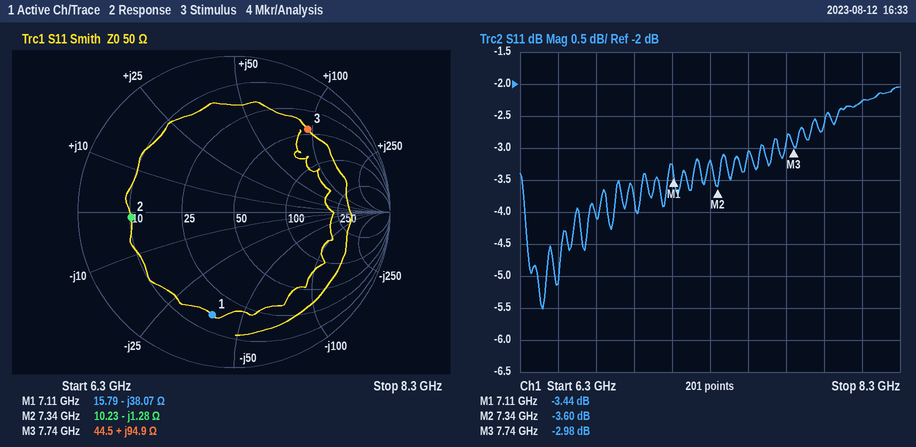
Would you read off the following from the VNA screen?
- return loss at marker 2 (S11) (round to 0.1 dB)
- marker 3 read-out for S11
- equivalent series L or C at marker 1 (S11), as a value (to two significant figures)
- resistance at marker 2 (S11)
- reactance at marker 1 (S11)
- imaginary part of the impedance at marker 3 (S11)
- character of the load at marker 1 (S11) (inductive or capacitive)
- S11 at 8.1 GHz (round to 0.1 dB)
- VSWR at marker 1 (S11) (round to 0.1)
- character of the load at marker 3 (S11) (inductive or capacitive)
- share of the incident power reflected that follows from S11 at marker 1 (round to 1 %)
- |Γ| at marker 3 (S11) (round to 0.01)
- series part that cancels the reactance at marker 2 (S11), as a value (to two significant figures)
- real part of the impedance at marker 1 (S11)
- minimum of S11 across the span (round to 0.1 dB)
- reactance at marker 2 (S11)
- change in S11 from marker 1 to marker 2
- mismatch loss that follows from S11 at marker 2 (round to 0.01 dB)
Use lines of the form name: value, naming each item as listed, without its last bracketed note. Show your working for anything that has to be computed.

return loss at marker 2 (S11): 3.6 dB
marker 3 read-out for S11: -2.98 dB
equivalent series L or C at marker 1 (S11), as a value: C = 1/(2π × 7.11 GHz × 38.07 Ω) ≈ 588 fF, so 590 fF to two significant figures
resistance at marker 2: 10.23 Ω
reactance at marker 1: -38.07 Ω
imaginary part of the impedance at marker 3: +94.9 Ω
character of the load at marker 1 (S11): capacitive
S11 at 8.1 GHz: -2.3 dB
VSWR at marker 1 (S11): 5.1
character of the load at marker 3 (S11): inductive
share of the incident power reflected that follows from S11 at marker 1: 10^(-3.44/10) ≈ 45 %
|Γ| at marker 3 (S11): 0.71
series part that cancels the reactance at marker 2 (S11), as a value: L = 1.28 Ω/(2π × 7.34 GHz) ≈ 28 pH
real part of the impedance at marker 1: 15.79 Ω
minimum of S11 across the span: -5.5 dB
reactance at marker 2: -1.28 Ω
change in S11 from marker 1 to marker 2: -3.6 − (-3.44) = -0.16 dB
mismatch loss that follows from S11 at marker 2: −10 log10(1 − 10^(-3.6/10)) ≈ 2.49 dB
